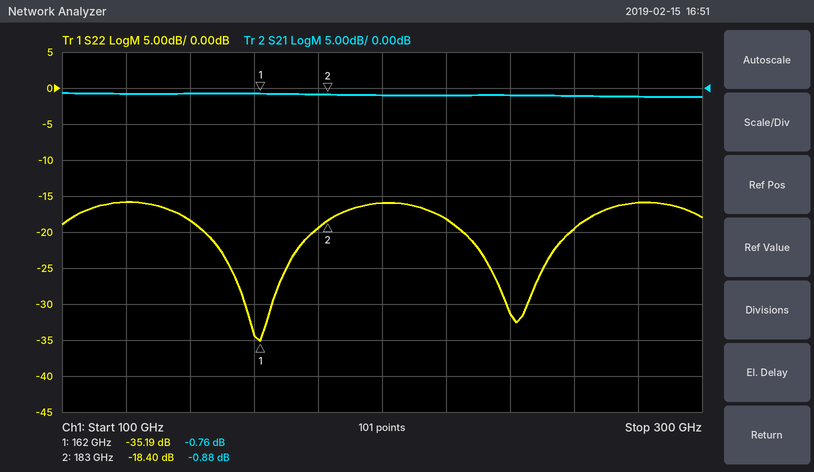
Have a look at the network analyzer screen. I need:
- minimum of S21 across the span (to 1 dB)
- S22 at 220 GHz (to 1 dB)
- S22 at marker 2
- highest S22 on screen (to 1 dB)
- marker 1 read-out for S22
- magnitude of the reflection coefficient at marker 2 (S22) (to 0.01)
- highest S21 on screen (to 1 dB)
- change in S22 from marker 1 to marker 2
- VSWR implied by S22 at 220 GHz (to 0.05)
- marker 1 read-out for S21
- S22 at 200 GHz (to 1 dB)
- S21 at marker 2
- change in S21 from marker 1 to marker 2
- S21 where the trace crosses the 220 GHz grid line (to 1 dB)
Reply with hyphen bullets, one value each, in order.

- -1 dB
- -18 dB
- -18.40 dB
- -16 dB
- -35.19 dB
- 0.12
- -1 dB
- 16.79 dB
- 1.30
- -0.76 dB
- -16 dB
- -0.88 dB
- -0.12 dB
- -1 dB
